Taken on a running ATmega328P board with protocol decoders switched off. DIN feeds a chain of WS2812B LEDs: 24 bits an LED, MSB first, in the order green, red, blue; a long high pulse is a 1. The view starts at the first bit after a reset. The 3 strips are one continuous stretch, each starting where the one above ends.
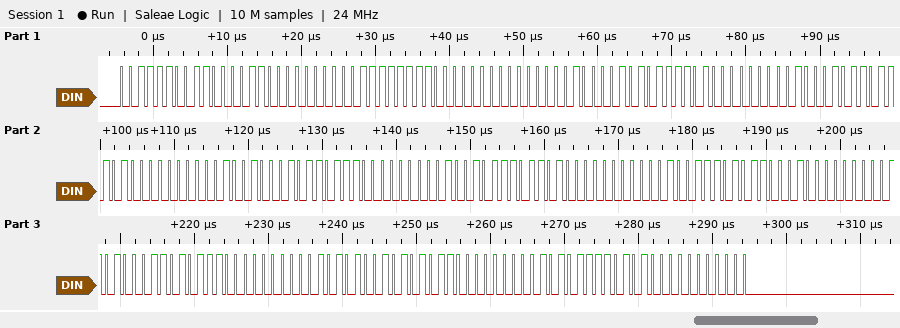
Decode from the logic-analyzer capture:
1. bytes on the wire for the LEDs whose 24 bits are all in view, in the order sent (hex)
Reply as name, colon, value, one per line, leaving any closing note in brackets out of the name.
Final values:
bytes on the wire for the LEDs whose 24 bits are all in view, in the order sent: 3C C3 00 3F C0 00 42 BD 00 45 BA 00 48 B7 00 4B B4 00 4E B1 00 51 AE 00 54 AB 00 57 A8 00
